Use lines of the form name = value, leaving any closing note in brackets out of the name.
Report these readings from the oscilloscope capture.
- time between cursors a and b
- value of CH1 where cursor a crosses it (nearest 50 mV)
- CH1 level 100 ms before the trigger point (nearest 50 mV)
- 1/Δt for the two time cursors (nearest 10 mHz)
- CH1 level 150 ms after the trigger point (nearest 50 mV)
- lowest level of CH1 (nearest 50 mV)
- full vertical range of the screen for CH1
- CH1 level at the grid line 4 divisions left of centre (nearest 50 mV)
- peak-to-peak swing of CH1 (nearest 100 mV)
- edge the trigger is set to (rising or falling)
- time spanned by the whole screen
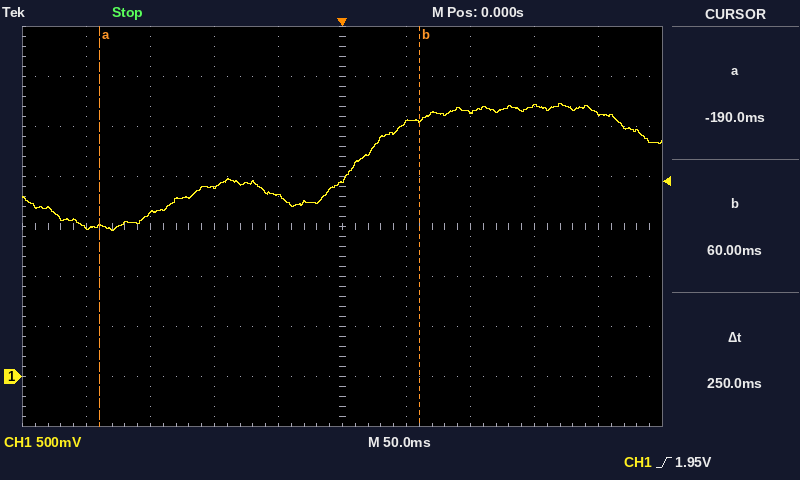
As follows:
time between cursors a and b = 250 ms
value of CH1 where cursor a crosses it = 1.50 V
CH1 level 100 ms before the trigger point = 1.90 V
1/Δt for the two time cursors = 4.00 Hz
CH1 level 150 ms after the trigger point = 2.70 V
lowest level of CH1 = 1.45 V
full vertical range of the screen for CH1 = 4 V
CH1 level at the grid line 4 divisions left of centre = 1.50 V
peak-to-peak swing of CH1 = 1.30 V
edge the trigger is set to = rising
time spanned by the whole screen = 500 ms
